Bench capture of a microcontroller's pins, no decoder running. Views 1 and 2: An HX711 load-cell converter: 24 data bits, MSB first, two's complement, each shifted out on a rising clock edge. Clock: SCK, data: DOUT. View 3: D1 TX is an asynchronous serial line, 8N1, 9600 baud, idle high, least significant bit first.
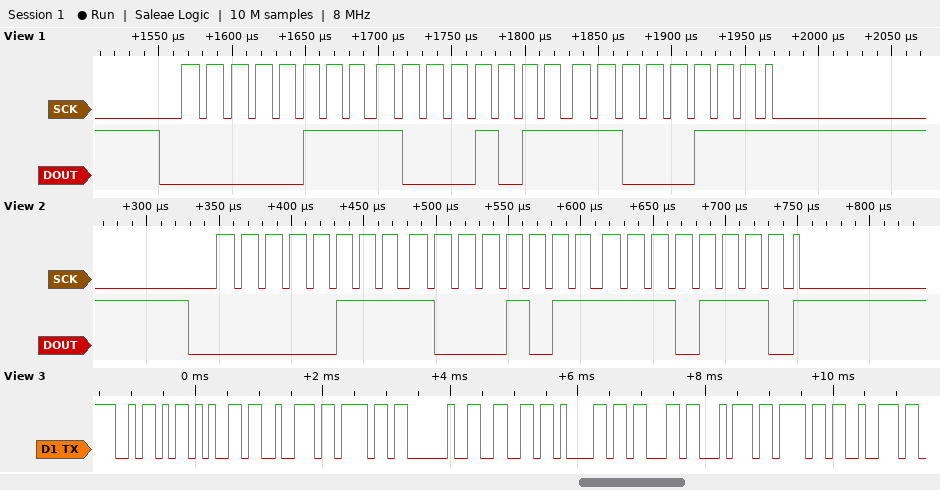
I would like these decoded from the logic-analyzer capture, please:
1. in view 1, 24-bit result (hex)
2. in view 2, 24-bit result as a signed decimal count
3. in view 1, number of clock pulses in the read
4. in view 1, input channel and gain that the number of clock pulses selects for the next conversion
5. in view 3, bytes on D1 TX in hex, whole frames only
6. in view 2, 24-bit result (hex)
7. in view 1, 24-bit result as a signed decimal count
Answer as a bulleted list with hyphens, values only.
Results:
- 0x078BC7
- 494574
- 25
- channel A, gain 128
- 5A 65 72 6F 20 66 61 63 74 6F 72
- 0x078BEE
- 494535
